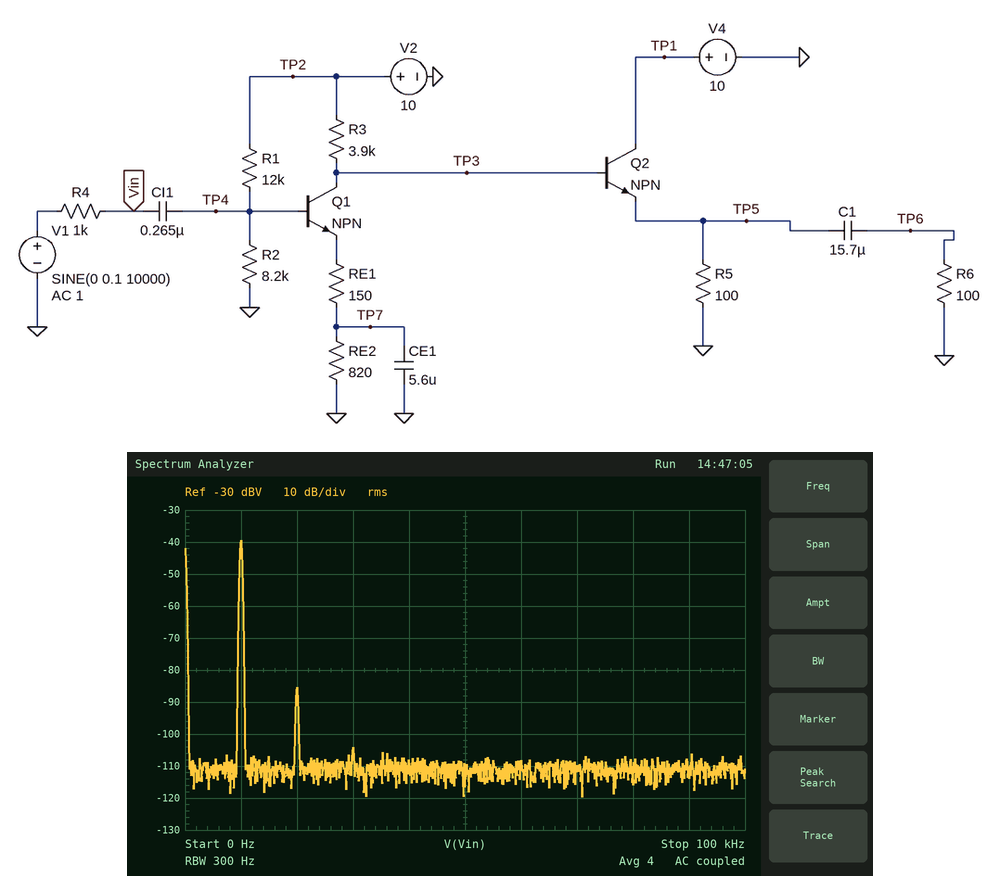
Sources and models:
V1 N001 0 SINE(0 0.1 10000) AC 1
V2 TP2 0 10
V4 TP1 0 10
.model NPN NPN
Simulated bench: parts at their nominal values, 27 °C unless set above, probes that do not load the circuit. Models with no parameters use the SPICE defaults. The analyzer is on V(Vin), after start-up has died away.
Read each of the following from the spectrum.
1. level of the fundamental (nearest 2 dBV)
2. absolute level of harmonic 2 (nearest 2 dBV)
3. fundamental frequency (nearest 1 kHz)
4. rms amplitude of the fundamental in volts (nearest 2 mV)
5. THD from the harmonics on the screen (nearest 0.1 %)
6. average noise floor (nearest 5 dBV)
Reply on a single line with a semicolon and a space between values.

-40 dBV; -86 dBV; 10 kHz; 10 mV; 0.5 %; -110 dBV
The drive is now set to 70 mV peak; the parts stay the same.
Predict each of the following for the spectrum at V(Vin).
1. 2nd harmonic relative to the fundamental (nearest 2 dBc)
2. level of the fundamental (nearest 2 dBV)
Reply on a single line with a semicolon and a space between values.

-50 dBc; -42 dBV
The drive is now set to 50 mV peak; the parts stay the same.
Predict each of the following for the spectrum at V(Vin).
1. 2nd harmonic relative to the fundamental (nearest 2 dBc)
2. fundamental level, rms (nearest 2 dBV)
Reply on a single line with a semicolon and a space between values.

-52 dBc; -46 dBV
